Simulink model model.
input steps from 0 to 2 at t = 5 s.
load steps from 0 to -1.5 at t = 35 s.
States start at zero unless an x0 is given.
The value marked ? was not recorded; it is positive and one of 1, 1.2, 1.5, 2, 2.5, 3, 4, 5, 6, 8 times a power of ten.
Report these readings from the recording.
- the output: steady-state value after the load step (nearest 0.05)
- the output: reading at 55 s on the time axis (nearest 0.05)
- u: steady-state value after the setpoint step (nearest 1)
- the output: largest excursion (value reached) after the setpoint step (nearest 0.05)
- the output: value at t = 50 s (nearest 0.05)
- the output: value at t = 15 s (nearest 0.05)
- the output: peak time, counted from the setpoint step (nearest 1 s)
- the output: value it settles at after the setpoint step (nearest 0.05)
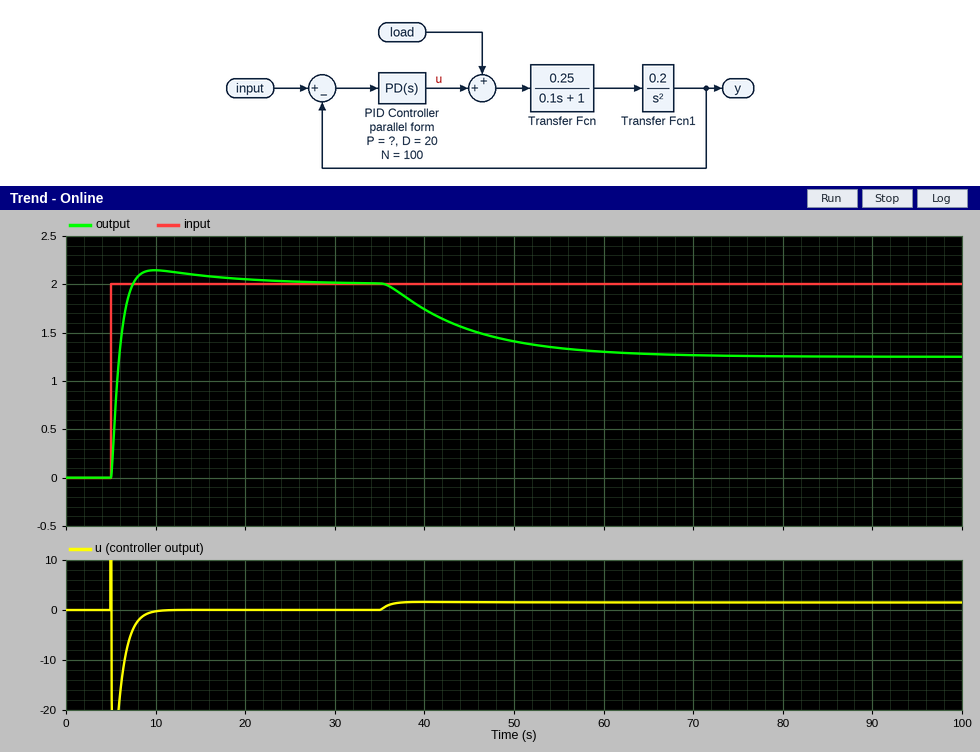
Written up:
1.25
1.35
0
2.15
1.40
2.10
5 s
2.00
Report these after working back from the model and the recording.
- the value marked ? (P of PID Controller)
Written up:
2
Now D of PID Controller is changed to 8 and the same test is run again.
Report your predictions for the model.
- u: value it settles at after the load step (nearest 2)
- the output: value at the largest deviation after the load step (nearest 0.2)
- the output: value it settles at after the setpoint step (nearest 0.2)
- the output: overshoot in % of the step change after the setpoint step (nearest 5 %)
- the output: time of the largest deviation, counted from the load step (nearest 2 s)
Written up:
2
1.2
2.0
25 %
12 s
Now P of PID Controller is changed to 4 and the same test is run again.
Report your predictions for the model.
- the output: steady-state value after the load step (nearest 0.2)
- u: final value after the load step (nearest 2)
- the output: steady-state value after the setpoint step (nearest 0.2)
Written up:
1.6
2
2.0
